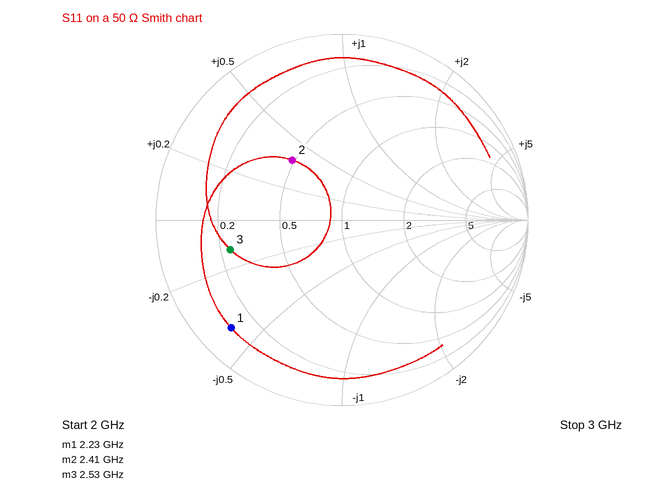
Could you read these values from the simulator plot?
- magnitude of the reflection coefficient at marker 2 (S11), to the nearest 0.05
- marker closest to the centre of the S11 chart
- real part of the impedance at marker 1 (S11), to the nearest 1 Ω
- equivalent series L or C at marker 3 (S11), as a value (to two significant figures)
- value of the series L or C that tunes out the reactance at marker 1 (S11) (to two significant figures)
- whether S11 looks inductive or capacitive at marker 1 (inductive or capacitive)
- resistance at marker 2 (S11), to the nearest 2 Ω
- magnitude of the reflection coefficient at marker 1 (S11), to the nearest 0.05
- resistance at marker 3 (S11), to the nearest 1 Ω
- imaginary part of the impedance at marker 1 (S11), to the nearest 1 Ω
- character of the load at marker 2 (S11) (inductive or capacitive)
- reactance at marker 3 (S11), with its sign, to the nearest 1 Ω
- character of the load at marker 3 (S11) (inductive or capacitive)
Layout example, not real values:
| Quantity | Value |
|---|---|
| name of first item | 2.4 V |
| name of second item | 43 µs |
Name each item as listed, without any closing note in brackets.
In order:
| Quantity | Value |
|---|---|
| magnitude of the reflection coefficient at marker 2 (S11), to the nearest 0.05 | 0.40 |
| marker closest to the centre of the S11 chart | marker 2 |
| real part of the impedance at marker 1 (S11), to the nearest 1 Ω | 5 Ω |
| equivalent series L or C at marker 3 (S11), as a value | 10 pF |
| value of the series L or C that tunes out the reactance at marker 1 (S11) | 1.4 nH |
| whether S11 looks inductive or capacitive at marker 1 | capacitive |
| resistance at marker 2 (S11), to the nearest 2 Ω | 24 Ω |
| magnitude of the reflection coefficient at marker 1 (S11), to the nearest 0.05 | 0.85 |
| resistance at marker 3 (S11), to the nearest 1 Ω | 12 Ω |
| imaginary part of the impedance at marker 1 (S11), to the nearest 1 Ω | -20 Ω |
| character of the load at marker 2 (S11) | inductive |
| reactance at marker 3 (S11), with its sign, to the nearest 1 Ω | -6 Ω |
| character of the load at marker 3 (S11) | capacitive |
